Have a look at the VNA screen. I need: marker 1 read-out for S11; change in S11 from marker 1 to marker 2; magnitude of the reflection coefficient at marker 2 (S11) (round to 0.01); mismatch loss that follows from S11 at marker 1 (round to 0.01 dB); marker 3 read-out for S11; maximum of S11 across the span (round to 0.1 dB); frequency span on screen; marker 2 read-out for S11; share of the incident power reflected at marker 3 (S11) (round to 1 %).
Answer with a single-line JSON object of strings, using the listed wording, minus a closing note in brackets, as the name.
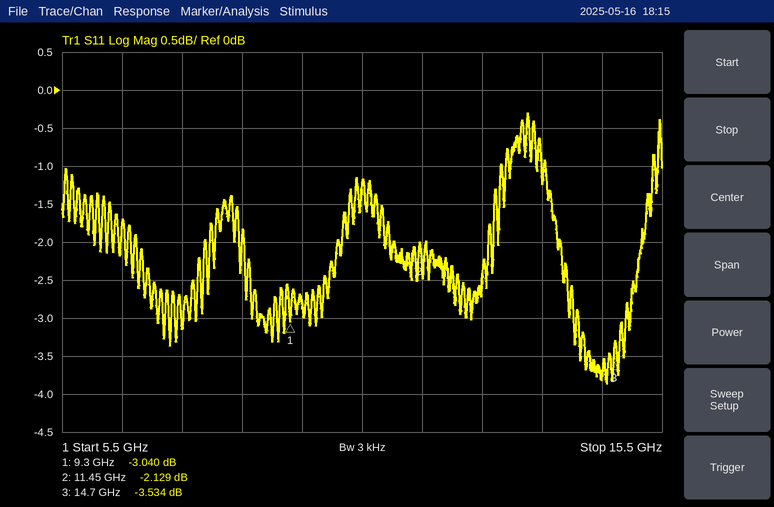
{"marker 1 read-out for S11": "-3.040 dB", "change in S11 from marker 1 to marker 2": "0.911 dB", "magnitude of the reflection coefficient at marker 2 (S11)": "0.78", "mismatch loss that follows from S11 at marker 1": "2.98 dB", "marker 3 read-out for S11": "-3.534 dB", "maximum of S11 across the span": "-0.3 dB", "frequency span on screen": "10 GHz", "marker 2 read-out for S11": "-2.129 dB", "share of the incident power reflected at marker 3 (S11)": "44 %"}
